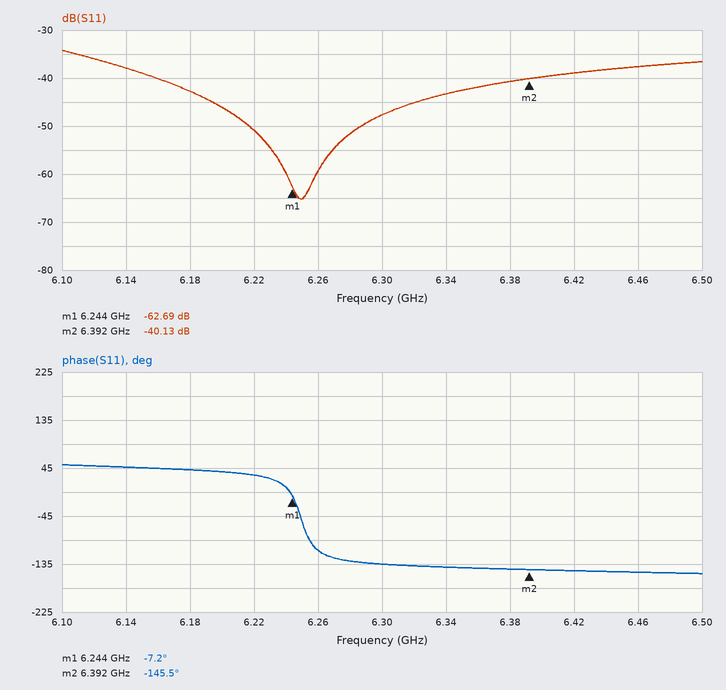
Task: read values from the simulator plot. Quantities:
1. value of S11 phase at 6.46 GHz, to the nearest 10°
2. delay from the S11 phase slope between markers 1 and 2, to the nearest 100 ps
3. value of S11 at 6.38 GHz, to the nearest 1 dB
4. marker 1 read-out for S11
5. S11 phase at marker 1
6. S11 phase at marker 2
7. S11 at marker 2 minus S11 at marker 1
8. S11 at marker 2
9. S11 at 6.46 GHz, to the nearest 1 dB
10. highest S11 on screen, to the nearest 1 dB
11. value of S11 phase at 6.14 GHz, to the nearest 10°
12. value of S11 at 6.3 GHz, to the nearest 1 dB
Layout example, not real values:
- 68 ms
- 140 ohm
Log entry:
- -150°
- 2.6 ns
- -41 dB
- -62.69 dB
- -7.2°
- -145.5°
- 22.56 dB
- -40.13 dB
- -38 dB
- -34 dB
- 50°
- -48 dB
